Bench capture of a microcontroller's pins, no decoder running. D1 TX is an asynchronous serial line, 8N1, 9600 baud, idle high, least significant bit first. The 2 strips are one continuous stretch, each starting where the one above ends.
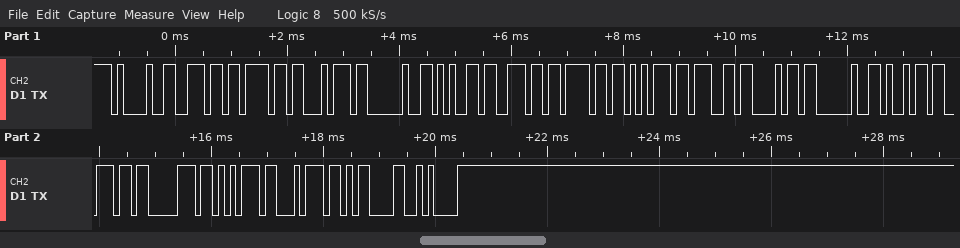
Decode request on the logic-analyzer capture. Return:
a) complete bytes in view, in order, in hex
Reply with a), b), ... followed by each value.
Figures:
a) 21 6E 6F 74 20 65 6E 6F 75 67 68 20 69 6E 70 75 74 0D 0A
